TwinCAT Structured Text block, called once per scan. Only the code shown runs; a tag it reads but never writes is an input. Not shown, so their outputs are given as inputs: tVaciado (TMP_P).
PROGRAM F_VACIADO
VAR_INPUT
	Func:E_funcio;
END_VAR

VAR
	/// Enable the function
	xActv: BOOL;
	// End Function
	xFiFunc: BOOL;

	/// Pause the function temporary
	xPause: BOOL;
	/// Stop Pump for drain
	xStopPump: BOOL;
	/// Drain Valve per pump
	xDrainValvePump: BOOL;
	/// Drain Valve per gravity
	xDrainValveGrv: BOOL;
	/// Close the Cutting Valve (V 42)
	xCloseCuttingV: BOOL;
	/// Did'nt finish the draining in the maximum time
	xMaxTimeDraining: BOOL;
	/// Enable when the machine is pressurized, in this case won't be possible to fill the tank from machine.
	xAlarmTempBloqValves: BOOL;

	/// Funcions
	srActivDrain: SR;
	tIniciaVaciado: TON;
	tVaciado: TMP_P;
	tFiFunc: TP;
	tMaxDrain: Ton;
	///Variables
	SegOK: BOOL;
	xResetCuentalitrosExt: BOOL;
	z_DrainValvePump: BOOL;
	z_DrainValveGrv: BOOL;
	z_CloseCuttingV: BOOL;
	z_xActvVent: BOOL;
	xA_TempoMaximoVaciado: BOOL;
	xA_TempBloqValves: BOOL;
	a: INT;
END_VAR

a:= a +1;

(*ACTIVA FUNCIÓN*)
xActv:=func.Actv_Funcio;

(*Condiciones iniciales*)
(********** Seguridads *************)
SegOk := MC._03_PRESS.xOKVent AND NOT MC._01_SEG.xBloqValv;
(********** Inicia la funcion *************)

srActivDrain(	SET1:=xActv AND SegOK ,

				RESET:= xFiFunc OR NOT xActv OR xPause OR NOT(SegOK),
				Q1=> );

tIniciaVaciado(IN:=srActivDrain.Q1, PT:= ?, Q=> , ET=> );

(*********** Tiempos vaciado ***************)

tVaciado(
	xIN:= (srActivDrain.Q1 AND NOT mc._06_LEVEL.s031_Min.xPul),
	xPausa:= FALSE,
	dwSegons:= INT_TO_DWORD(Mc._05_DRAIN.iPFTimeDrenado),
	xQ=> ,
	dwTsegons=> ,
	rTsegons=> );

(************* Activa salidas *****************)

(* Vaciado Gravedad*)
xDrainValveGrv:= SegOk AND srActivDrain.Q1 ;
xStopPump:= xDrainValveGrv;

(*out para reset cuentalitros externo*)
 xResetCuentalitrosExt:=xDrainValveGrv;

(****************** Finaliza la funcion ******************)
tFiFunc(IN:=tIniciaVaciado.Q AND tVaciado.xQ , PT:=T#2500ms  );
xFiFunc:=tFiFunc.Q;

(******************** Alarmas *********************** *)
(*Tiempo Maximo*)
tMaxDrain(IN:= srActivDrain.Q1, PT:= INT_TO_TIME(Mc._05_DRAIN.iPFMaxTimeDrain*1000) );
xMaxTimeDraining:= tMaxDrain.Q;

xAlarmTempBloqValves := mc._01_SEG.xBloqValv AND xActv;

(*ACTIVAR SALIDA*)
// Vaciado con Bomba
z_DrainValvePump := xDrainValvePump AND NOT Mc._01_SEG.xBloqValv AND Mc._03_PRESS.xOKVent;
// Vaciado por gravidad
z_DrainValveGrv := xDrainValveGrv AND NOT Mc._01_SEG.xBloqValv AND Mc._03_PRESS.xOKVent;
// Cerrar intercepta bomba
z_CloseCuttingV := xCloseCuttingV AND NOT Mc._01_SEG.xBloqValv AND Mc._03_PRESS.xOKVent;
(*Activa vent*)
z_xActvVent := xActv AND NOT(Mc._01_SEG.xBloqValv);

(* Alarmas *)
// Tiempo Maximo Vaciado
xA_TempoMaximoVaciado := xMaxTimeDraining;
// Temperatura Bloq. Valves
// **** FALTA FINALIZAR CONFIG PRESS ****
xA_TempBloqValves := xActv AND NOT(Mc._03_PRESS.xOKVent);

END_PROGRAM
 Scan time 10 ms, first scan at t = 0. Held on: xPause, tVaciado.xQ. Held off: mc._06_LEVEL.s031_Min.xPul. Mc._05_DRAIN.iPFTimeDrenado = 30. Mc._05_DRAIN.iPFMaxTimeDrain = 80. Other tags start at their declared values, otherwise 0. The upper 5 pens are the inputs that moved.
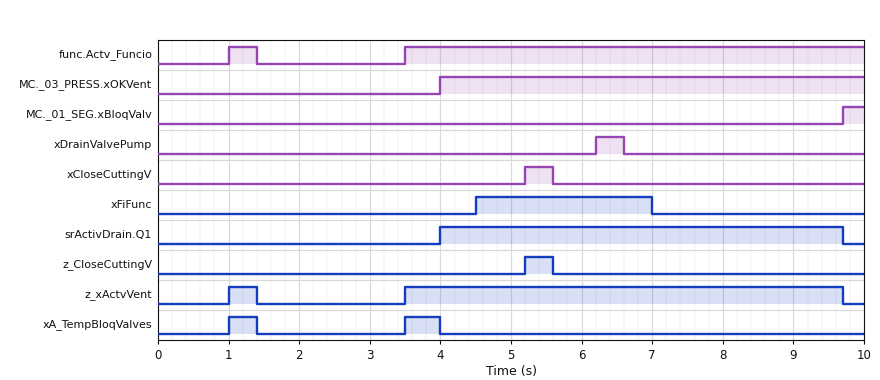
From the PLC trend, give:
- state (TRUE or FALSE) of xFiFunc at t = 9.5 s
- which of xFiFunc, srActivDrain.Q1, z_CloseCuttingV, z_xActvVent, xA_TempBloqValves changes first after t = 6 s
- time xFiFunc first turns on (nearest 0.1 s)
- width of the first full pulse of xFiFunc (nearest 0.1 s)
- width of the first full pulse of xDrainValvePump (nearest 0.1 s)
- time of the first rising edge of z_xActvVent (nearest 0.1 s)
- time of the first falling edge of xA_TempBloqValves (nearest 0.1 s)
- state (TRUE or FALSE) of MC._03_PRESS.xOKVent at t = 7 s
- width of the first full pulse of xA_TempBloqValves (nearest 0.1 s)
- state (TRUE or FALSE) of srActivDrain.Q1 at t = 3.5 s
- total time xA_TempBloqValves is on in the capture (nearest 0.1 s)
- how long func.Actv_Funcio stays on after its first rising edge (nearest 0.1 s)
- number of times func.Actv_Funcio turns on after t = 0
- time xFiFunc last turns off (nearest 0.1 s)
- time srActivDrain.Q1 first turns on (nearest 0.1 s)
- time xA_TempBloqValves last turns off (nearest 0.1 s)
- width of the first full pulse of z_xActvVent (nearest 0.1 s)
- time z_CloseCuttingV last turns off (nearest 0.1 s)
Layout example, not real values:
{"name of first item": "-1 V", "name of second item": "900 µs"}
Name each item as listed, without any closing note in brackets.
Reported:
{"state (TRUE or FALSE) of xFiFunc at t = 9.5 s": "FALSE", "which of xFiFunc, srActivDrain.Q1, z_CloseCuttingV, z_xActvVent, xA_TempBloqValves changes first after t = 6 s": "xFiFunc", "time xFiFunc first turns on": "4.5 s", "width of the first full pulse of xFiFunc": "2.5 s", "width of the first full pulse of xDrainValvePump": "0.4 s", "time of the first rising edge of z_xActvVent": "1.0 s", "time of the first falling edge of xA_TempBloqValves": "1.4 s", "state (TRUE or FALSE) of MC._03_PRESS.xOKVent at t = 7 s": "TRUE", "width of the first full pulse of xA_TempBloqValves": "0.4 s", "state (TRUE or FALSE) of srActivDrain.Q1 at t = 3.5 s": "FALSE", "total time xA_TempBloqValves is on in the capture": "0.9 s", "how long func.Actv_Funcio stays on after its first rising edge": "0.4 s", "number of times func.Actv_Funcio turns on after t = 0": "2", "time xFiFunc last turns off": "7.0 s", "time srActivDrain.Q1 first turns on": "4.0 s", "time xA_TempBloqValves last turns off": "4.0 s", "width of the first full pulse of z_xActvVent": "0.4 s", "time z_CloseCuttingV last turns off": "5.6 s"}
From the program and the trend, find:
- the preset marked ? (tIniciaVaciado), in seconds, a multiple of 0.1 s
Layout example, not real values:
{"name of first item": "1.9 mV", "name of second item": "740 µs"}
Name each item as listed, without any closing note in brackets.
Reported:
{"the preset marked ? (tIniciaVaciado), in seconds, a multiple of 0.1 s": "0.5 s"}
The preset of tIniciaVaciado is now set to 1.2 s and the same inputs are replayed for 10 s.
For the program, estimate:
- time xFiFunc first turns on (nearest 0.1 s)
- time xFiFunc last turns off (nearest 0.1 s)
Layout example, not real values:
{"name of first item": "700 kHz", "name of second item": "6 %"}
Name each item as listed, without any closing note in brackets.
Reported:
{"time xFiFunc first turns on": "5.2 s", "time xFiFunc last turns off": "7.7 s"}
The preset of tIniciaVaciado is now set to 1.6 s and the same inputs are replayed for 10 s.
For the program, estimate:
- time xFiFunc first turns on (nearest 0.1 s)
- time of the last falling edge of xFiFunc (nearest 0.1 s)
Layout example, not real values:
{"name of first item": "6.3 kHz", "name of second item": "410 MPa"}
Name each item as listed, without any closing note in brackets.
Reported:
{"time xFiFunc first turns on": "5.6 s", "time of the last falling edge of xFiFunc": "8.1 s"}
